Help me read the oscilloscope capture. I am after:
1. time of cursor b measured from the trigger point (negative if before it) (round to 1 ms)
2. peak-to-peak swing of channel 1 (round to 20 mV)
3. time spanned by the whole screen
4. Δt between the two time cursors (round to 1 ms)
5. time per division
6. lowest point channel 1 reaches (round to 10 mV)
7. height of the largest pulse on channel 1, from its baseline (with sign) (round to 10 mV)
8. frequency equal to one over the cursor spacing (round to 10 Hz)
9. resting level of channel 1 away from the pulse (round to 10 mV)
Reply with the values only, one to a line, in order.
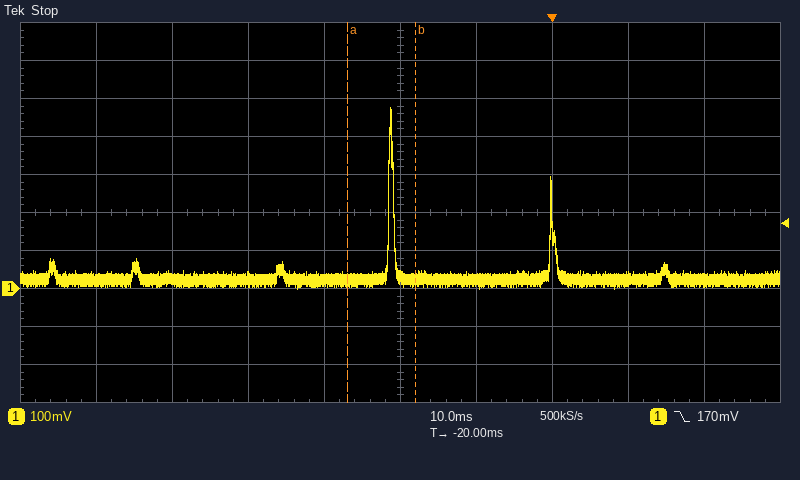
-18 ms
480 mV
100 ms
9 ms
10 ms
0 mV
+450 mV
110 Hz
20 mV
